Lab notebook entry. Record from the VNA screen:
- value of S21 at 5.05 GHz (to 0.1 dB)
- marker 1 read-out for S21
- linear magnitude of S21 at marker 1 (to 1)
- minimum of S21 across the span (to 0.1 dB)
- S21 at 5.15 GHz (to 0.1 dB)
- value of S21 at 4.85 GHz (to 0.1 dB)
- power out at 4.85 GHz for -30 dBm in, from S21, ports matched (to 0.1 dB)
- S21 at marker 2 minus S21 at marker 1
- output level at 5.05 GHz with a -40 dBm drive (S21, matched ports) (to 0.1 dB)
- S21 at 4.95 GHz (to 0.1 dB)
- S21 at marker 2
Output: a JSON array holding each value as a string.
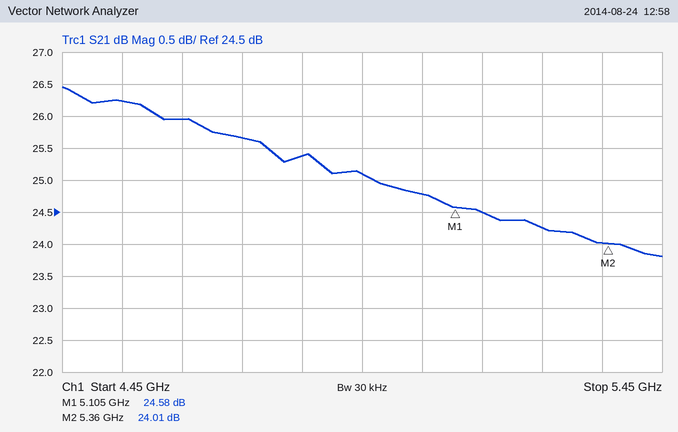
["24.8 dB", "24.58 dB", "17", "23.8 dB", "24.5 dB", "25.4 dB", "-4.6 dBm", "-0.57 dB", "-15.2 dBm", "25.1 dB", "24.01 dB"]
